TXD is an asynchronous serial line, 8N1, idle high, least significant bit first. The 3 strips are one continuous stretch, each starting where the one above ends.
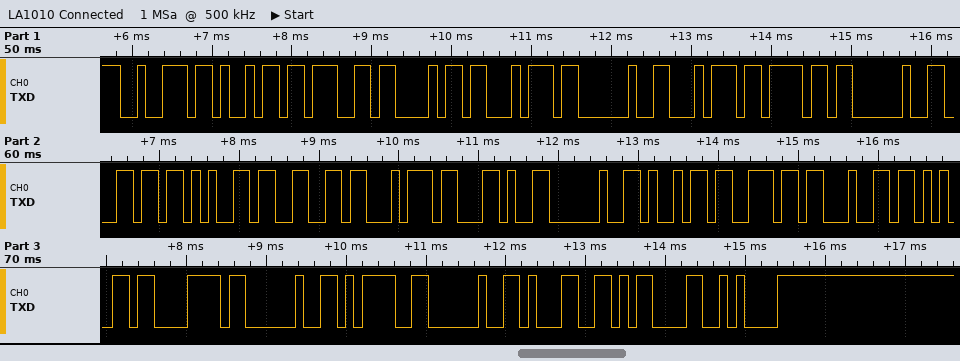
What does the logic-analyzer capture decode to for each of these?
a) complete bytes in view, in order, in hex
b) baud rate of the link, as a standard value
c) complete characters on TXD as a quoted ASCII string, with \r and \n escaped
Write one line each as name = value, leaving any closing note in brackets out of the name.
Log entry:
complete bytes in view, in order, in hex = 72 69 67 68 74 20 74 6F 20 6C 65 66 74 2C 20 69 6E 64 65 78 20 3D 20 31 0D 0A
baud rate of the link, as a standard value = 9600 baud
complete characters on TXD as a quoted ASCII string, with \r and \n escaped = "right to left, index = 1\r\n"
